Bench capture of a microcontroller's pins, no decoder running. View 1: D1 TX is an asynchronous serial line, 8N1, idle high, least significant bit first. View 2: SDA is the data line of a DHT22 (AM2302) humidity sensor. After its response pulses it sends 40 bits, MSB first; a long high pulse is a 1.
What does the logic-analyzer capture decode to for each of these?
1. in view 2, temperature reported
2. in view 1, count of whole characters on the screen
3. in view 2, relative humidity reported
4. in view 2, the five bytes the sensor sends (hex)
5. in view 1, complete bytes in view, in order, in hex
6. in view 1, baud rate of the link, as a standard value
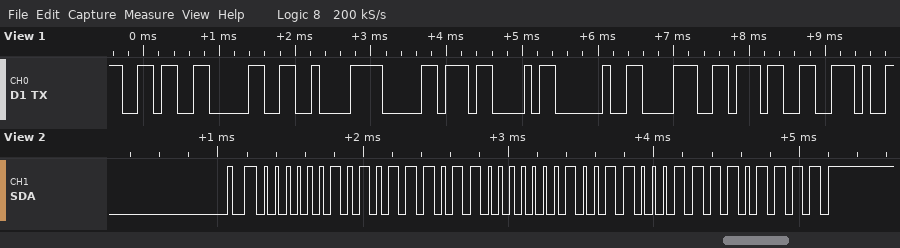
30.5 °C
9
69.9 %
02 BB 01 31 EF
0x36 0x30 0xC2 0xB0 0x43 0x20 0x38 0x37 0x2E
9600 baud
